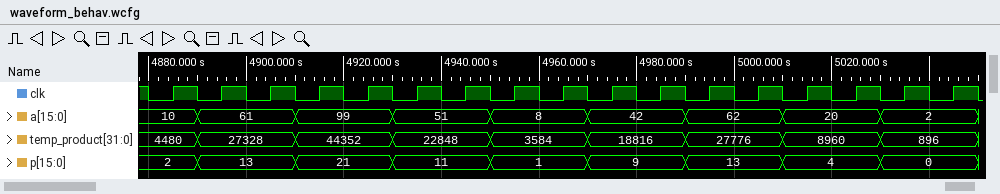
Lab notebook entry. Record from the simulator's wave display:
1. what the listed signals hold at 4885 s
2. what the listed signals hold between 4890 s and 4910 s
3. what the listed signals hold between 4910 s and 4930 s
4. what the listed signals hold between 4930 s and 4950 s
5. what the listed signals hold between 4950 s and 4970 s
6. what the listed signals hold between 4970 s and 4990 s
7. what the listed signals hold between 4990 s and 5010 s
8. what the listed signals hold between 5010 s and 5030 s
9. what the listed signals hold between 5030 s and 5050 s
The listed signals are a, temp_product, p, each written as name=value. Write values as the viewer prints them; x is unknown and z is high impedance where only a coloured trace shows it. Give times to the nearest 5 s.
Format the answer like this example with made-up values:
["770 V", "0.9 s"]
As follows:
["a=10, temp_product=4480, p=2", "a=61, temp_product=27328, p=13", "a=99, temp_product=44352, p=21", "a=51, temp_product=22848, p=11", "a=8, temp_product=3584, p=1", "a=42, temp_product=18816, p=9", "a=62, temp_product=27776, p=13", "a=20, temp_product=8960, p=4", "a=2, temp_product=896, p=0"]
